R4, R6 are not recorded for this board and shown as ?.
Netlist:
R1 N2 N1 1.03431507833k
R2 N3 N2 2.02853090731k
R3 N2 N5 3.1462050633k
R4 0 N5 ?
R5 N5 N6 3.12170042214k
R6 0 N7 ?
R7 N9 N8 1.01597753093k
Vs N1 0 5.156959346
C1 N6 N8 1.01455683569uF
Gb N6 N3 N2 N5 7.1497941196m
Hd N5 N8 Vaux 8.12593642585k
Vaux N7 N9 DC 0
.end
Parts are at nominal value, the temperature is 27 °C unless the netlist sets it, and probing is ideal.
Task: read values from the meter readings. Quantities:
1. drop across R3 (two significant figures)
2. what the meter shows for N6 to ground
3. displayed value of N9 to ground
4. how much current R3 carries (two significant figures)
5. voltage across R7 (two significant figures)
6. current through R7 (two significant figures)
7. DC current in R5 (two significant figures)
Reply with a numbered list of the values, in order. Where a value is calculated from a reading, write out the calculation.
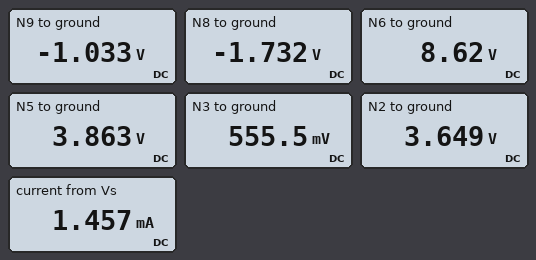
1. 3.863 V - 3.649 V = 210 mV
2. 8.62 V
3. -1.033 V
4. (3.863 V - 3.649 V) / 3.146 kΩ = 68 µA
5. -1.033 V - (-1.732 V) = 700 mV
6. (-1.033 V - (-1.732 V)) / 1.016 kΩ = 690 µA
7. (8.62 V - 3.863 V) / 3.122 kΩ = 1.5 mA
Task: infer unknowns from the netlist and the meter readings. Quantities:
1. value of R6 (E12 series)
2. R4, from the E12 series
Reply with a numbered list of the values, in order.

1. 1.5 kΩ
2. 1.8 kΩ
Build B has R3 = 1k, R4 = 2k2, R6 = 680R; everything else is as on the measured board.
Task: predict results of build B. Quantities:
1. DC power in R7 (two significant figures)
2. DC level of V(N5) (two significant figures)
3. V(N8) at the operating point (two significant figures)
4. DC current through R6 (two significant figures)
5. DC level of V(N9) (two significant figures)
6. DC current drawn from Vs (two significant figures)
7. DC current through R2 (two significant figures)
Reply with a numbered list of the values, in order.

1. 410 µW
2. 4.1 V
3. -1.1 V
4. 640 µA
5. -430 mV
6. 1.2 mA
7. 1.4 mA
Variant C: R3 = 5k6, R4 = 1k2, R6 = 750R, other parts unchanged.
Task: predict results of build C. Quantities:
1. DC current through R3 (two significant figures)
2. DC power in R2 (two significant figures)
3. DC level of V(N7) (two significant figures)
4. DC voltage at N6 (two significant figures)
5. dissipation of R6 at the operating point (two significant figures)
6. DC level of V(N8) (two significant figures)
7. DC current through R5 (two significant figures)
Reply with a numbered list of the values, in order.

1. 56 µA
2. 10 mW
3. -380 mV
4. 10 V
5. 190 µW
6. -890 mV
7. 2.2 mA
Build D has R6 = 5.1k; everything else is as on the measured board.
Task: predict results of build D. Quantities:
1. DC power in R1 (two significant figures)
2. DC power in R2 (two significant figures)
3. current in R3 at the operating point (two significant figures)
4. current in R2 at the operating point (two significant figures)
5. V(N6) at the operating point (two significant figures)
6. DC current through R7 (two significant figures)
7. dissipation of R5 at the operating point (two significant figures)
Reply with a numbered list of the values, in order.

1. 84 µW
2. 180 µW
3. 13 µA
4. 300 µA
5. 5.8 V
6. 2.4 mA
7. 280 µW
